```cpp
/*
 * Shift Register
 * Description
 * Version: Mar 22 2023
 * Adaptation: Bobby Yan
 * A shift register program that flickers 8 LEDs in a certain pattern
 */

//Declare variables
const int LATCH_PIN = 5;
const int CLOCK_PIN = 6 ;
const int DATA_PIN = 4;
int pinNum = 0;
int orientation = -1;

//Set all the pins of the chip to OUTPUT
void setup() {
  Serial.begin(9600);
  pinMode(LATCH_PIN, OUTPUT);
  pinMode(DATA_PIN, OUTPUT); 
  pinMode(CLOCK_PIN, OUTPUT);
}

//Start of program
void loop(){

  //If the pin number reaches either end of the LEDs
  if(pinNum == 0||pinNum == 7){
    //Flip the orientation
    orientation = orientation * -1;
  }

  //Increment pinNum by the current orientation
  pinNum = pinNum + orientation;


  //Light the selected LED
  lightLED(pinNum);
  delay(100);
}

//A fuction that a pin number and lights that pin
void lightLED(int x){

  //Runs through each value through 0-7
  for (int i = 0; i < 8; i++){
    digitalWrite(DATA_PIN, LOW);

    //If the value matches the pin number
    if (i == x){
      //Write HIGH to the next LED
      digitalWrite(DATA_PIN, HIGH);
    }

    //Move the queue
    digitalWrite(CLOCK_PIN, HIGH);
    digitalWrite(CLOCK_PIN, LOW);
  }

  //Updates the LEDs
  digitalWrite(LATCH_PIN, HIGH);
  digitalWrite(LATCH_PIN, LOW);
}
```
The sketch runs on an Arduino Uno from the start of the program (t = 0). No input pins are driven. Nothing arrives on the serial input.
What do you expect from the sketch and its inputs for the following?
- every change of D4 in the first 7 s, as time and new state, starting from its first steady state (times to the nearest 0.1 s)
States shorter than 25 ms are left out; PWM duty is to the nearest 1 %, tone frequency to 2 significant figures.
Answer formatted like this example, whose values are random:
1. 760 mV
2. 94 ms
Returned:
1. 0 s low; 0.6 s high; 0.7 s low; 2 s high; 2.1 s low; 3.4 s high; 3.5 s low; 4.8 s high; 4.9 s low; 6.2 s high; 6.3 s low
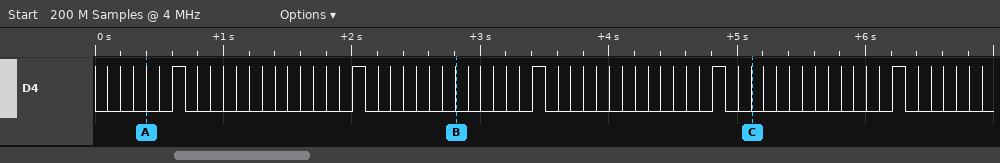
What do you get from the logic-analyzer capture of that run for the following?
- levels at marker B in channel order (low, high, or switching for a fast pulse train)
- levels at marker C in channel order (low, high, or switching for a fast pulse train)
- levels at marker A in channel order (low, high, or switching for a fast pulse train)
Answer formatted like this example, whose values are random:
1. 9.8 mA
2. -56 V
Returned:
1. D4 low
2. D4 low
3. D4 low
